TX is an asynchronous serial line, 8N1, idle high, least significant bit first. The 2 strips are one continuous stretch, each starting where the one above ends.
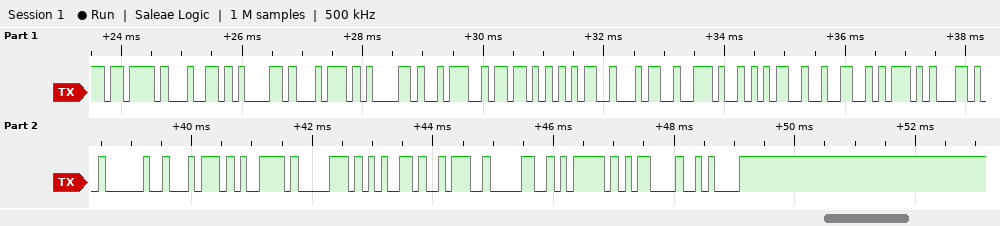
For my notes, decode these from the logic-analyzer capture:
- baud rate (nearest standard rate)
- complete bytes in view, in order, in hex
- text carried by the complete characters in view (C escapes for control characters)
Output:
9600 baud
7B 64 61 74 61 3A 5B 35 34 2E 35 32 5D 2C 20 74 79 70 65 3A 30 7D 0D 0A
"{data:[54.52], type:0}\r\n"
